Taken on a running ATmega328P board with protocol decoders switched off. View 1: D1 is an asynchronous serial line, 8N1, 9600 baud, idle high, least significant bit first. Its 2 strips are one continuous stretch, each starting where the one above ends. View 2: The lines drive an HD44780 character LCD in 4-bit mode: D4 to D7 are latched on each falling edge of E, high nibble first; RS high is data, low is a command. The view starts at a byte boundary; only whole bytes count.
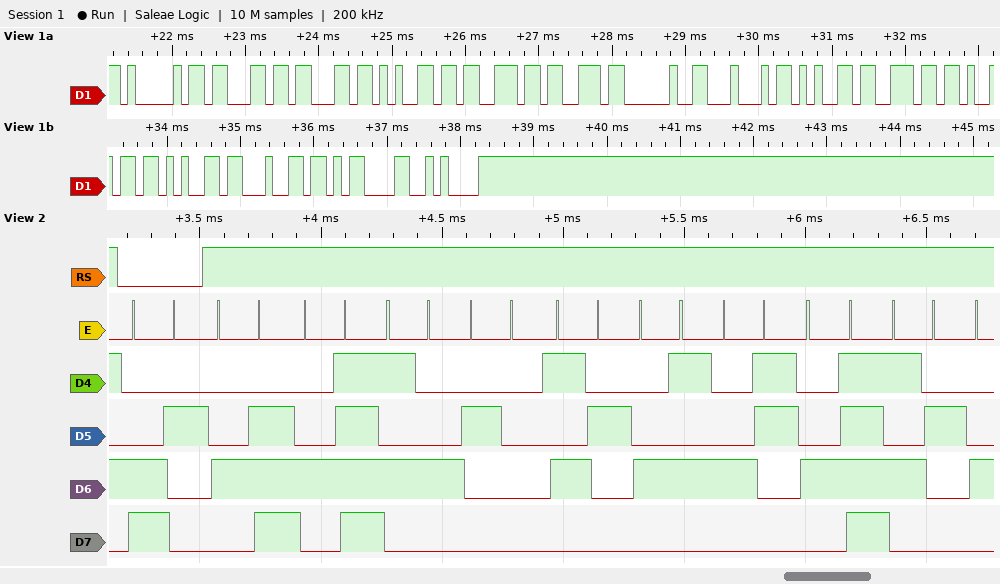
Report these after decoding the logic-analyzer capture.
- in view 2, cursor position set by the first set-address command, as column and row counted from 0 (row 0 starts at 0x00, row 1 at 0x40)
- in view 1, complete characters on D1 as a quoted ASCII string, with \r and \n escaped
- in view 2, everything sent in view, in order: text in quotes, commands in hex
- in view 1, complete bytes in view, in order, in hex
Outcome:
column 2, row 1
"Access Denied\r\n"
0xC2 "NOT RECOR"
41 63 63 65 73 73 20 44 65 6E 69 65 64 0D 0A
